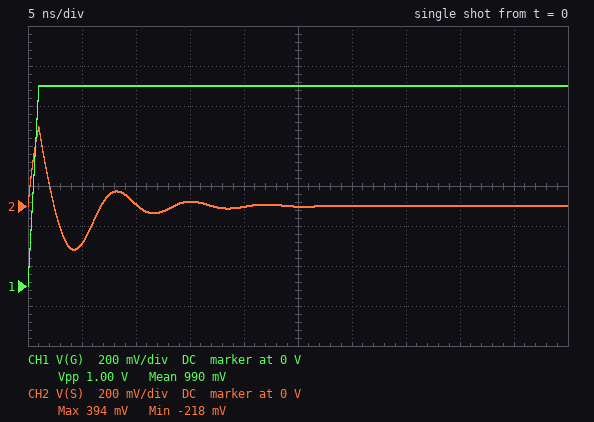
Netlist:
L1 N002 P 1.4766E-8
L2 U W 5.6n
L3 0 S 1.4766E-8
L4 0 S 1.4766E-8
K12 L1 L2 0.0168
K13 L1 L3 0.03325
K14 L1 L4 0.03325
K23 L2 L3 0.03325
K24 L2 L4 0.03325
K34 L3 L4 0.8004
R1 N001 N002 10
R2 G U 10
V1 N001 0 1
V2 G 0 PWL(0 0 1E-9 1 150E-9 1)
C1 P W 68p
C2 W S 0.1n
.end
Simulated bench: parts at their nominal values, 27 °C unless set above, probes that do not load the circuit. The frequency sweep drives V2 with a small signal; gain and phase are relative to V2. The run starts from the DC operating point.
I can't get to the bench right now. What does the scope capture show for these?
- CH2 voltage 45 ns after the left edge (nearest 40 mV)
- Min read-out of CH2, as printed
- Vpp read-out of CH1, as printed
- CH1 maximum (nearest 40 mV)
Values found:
0 V
-218 mV
1.00 V
1.00 V
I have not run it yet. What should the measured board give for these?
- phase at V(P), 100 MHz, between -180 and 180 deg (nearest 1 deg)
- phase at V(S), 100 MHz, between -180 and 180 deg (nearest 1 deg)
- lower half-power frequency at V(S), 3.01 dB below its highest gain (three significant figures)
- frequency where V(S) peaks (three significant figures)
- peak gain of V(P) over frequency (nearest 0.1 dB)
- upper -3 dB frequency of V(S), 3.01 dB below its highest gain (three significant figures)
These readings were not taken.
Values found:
31 deg
111 deg
118 MHz
145 MHz
-4.5 dB
182 MHz
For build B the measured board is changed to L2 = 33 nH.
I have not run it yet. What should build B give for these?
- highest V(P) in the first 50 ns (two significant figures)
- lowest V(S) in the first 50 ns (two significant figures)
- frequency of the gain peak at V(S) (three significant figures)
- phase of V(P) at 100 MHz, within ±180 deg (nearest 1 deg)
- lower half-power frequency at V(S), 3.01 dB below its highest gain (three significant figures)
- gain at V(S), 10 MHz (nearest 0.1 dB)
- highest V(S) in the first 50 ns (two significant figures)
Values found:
1.2 V
-97 mV
144 MHz
-34 deg
61.4 MHz
-46.0 dB
170 mV
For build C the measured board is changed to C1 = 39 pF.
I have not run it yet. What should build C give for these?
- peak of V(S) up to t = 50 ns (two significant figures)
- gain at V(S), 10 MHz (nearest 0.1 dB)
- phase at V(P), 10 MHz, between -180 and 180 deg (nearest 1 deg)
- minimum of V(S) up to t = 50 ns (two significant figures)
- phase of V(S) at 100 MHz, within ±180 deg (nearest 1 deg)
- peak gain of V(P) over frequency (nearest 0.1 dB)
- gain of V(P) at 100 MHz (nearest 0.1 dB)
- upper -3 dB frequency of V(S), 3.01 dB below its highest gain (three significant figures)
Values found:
400 mV
-45.7 dB
89 deg
-260 mV
109 deg
-2.1 dB
-12.0 dB
198 MHz
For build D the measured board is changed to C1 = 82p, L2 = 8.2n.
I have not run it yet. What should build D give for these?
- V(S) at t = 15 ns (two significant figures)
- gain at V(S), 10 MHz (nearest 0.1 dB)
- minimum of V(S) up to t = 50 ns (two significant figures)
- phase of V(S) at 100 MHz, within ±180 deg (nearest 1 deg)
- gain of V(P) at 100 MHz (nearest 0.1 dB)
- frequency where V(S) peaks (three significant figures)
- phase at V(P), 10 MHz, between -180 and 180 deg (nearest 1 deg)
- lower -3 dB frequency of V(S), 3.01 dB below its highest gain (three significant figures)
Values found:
19 mV
-45.8 dB
-200 mV
106 deg
-6.9 dB
140 MHz
86 deg
115 MHz
